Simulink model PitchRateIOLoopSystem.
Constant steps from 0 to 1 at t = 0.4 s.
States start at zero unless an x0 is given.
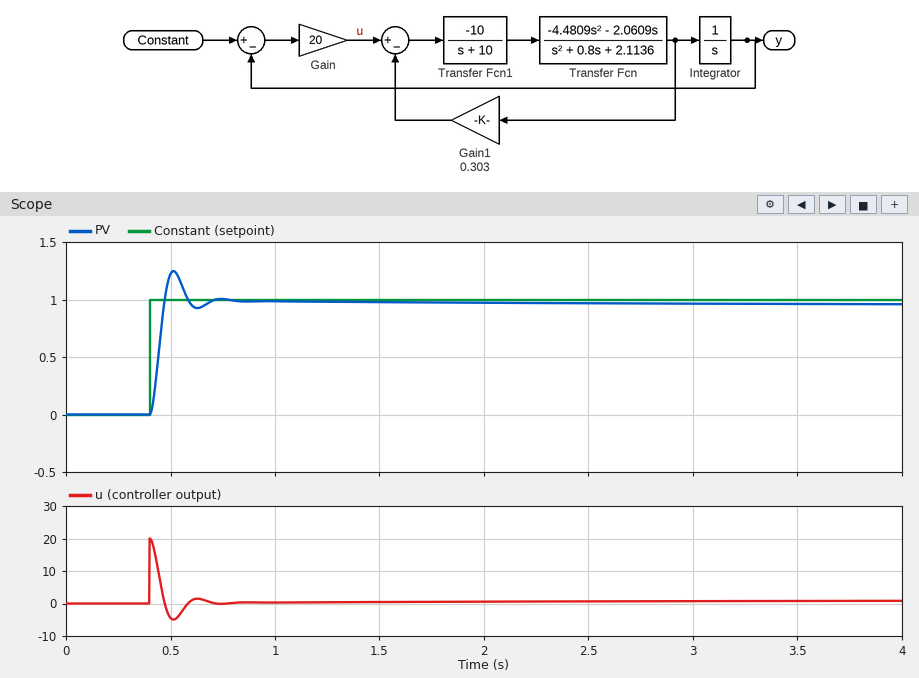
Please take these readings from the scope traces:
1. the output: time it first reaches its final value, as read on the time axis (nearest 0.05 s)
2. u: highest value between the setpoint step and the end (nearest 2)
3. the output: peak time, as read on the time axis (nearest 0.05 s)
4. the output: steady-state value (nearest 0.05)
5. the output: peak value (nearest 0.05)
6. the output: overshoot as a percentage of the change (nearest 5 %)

0.45 s
20
0.50 s
0.95
1.25
30 %
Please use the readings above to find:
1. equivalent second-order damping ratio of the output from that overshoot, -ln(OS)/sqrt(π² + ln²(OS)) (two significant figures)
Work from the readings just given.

0.36
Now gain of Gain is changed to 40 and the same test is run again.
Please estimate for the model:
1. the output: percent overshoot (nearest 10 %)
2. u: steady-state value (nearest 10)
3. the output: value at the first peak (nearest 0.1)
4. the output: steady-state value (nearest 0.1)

40 %
0
1.4
1.0
